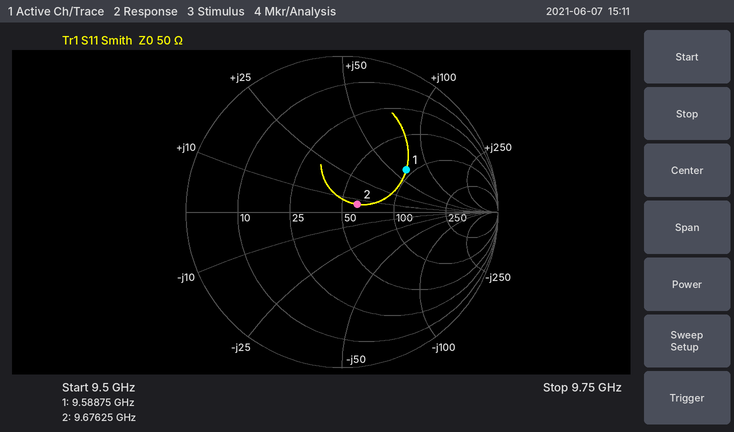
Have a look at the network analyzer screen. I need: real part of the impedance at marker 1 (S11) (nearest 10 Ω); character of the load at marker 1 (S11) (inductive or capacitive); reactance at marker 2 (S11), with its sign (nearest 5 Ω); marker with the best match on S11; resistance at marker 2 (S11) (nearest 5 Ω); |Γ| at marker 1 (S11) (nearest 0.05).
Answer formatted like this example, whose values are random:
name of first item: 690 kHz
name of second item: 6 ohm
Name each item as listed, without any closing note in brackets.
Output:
real part of the impedance at marker 1 (S11): 90 Ω
character of the load at marker 1 (S11): inductive
reactance at marker 2 (S11), with its sign: +5 Ω
marker with the best match on S11: marker 2
resistance at marker 2 (S11): 60 Ω
|Γ| at marker 1 (S11): 0.50
